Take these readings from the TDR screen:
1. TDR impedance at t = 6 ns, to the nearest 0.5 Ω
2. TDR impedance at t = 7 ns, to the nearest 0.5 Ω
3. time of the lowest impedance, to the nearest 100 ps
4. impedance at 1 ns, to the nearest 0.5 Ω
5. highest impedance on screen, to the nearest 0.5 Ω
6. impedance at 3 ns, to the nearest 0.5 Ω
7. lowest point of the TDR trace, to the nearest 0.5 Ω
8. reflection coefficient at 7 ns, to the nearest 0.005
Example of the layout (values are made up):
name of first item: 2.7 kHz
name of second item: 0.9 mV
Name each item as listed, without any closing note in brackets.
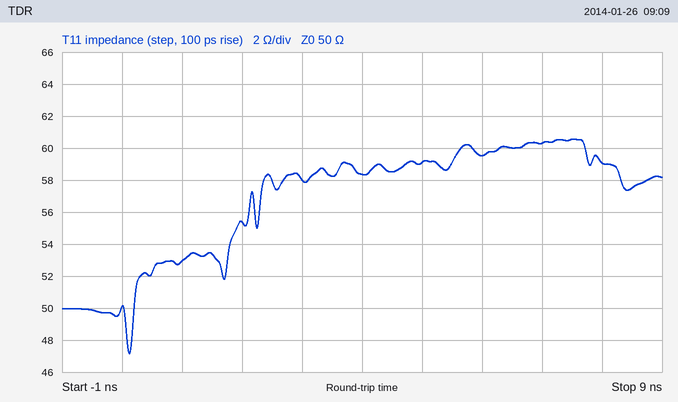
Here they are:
TDR impedance at t = 6 ns, to the nearest 0.5 Ω: 59.5 Ω
TDR impedance at t = 7 ns, to the nearest 0.5 Ω: 60.5 Ω
time of the lowest impedance, to the nearest 100 ps: 100 ps
impedance at 1 ns, to the nearest 0.5 Ω: 53.0 Ω
highest impedance on screen, to the nearest 0.5 Ω: 60.5 Ω
impedance at 3 ns, to the nearest 0.5 Ω: 58.0 Ω
lowest point of the TDR trace, to the nearest 0.5 Ω: 47.0 Ω
reflection coefficient at 7 ns, to the nearest 0.005: +0.095
